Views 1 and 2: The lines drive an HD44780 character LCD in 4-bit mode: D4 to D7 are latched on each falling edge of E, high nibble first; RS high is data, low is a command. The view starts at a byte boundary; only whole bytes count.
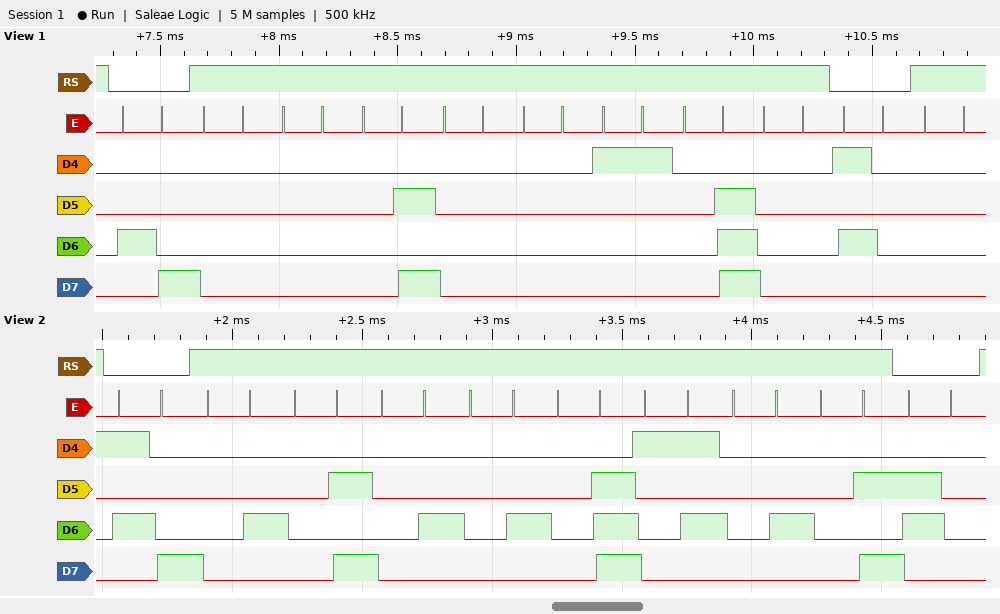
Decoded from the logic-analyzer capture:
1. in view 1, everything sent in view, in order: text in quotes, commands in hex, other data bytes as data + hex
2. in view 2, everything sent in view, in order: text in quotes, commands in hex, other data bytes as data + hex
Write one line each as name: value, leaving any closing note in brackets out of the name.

in view 1, everything sent in view, in order: text in quotes, commands in hex, other data bytes as data + hex: 0x48 data 00 00 0A 00 00 11 0E 00 0x50 data 00
in view 2, everything sent in view, in order: text in quotes, commands in hex, other data bytes as data + hex: 0x58 data 04 0A 04 04 0E 15 04 0A 0x60
